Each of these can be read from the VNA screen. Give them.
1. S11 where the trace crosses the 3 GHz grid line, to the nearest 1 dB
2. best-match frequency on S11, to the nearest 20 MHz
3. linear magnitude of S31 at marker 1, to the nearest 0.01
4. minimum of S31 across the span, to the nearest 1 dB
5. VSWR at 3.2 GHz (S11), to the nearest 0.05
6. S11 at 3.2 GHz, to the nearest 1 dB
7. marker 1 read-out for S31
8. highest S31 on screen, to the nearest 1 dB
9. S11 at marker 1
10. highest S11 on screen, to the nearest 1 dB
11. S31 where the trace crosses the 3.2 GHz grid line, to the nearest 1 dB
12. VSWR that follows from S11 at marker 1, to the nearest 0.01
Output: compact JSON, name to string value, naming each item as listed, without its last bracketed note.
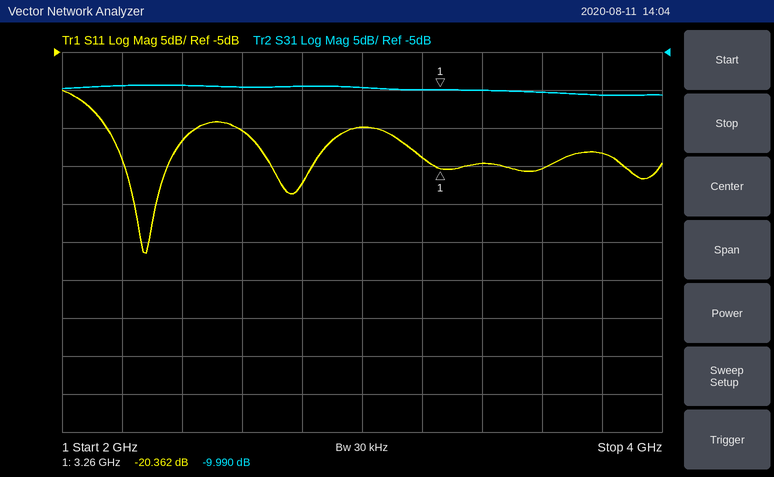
{"S11 where the trace crosses the 3 GHz grid line, to the nearest 1 dB": "-15 dB", "best-match frequency on S11, to the nearest 20 MHz": "2.28 GHz", "linear magnitude of S31 at marker 1, to the nearest 0.01": "0.32", "minimum of S31 across the span, to the nearest 1 dB": "-11 dB", "VSWR at 3.2 GHz (S11), to the nearest 0.05": "1.25", "S11 at 3.2 GHz, to the nearest 1 dB": "-19 dB", "marker 1 read-out for S31": "-9.990 dB", "highest S31 on screen, to the nearest 1 dB": "-9 dB", "S11 at marker 1": "-20.362 dB", "highest S11 on screen, to the nearest 1 dB": "-10 dB", "S31 where the trace crosses the 3.2 GHz grid line, to the nearest 1 dB": "-10 dB", "VSWR that follows from S11 at marker 1, to the nearest 0.01": "1.21"}
